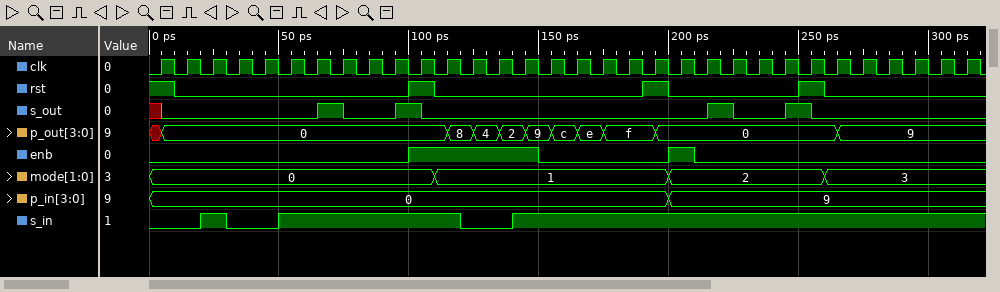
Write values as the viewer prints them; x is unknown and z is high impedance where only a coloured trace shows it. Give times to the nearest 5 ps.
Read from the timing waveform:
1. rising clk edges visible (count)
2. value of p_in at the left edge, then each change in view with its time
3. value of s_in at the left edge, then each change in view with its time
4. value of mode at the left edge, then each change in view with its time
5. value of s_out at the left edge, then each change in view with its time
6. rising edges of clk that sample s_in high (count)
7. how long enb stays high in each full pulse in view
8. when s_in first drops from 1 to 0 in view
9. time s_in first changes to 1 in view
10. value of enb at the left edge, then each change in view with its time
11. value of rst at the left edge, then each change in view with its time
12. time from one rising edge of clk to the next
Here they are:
32
0, 9 at 200 ps
0, 1 at 20 ps, 0 at 30 ps, 1 at 50 ps, 0 at 120 ps, 1 at 140 ps
0, 1 at 110 ps, 2 at 200 ps, 3 at 260 ps
x, 0 at 5 ps, 1 at 65 ps, 0 at 75 ps, 1 at 95 ps, 0 at 105 ps, 1 at 215 ps, 0 at 225 ps, 1 at 245 ps, 0 at 255 ps
26
50 ps, 10 ps
30 ps
20 ps
0, 1 at 100 ps, 0 at 150 ps, 1 at 200 ps, 0 at 210 ps
1, 0 at 10 ps, 1 at 100 ps, 0 at 110 ps, 1 at 190 ps, 0 at 200 ps, 1 at 250 ps, 0 at 260 ps
10 ps
